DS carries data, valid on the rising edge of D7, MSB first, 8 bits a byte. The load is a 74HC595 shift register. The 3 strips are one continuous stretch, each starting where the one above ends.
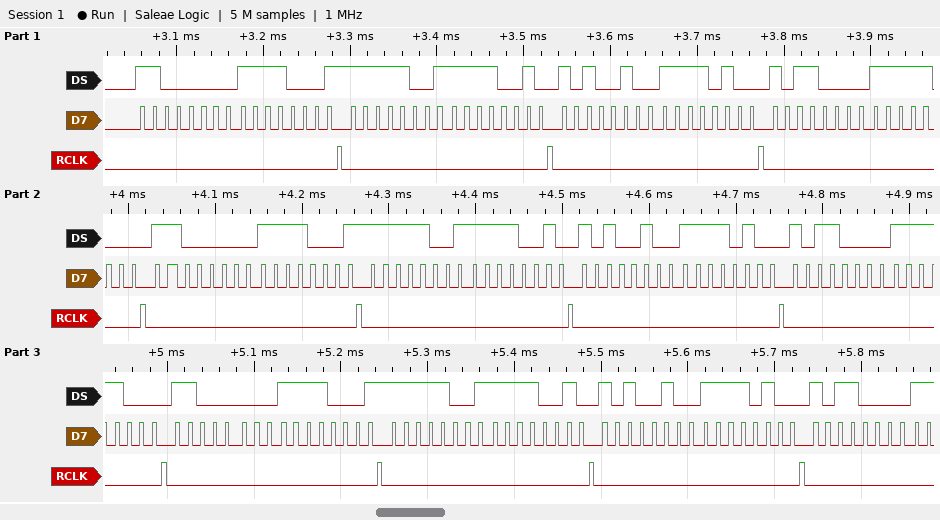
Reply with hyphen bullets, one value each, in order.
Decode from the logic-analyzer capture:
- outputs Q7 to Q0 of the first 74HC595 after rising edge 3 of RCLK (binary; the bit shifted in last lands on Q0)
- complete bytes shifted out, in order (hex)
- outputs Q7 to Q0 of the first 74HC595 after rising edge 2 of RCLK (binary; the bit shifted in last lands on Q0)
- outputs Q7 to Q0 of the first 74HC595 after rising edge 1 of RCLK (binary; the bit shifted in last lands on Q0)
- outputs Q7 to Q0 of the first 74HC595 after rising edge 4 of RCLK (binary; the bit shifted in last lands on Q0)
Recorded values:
- 11110100
- C0 F1 F9 F2 A4 F4 B0 F8 C0 F1 F9 F2 A4 F4 B0 F8 C0 F1 F9 F2 A4 F4 B0
- 11110010
- 11110001
- 11111000
